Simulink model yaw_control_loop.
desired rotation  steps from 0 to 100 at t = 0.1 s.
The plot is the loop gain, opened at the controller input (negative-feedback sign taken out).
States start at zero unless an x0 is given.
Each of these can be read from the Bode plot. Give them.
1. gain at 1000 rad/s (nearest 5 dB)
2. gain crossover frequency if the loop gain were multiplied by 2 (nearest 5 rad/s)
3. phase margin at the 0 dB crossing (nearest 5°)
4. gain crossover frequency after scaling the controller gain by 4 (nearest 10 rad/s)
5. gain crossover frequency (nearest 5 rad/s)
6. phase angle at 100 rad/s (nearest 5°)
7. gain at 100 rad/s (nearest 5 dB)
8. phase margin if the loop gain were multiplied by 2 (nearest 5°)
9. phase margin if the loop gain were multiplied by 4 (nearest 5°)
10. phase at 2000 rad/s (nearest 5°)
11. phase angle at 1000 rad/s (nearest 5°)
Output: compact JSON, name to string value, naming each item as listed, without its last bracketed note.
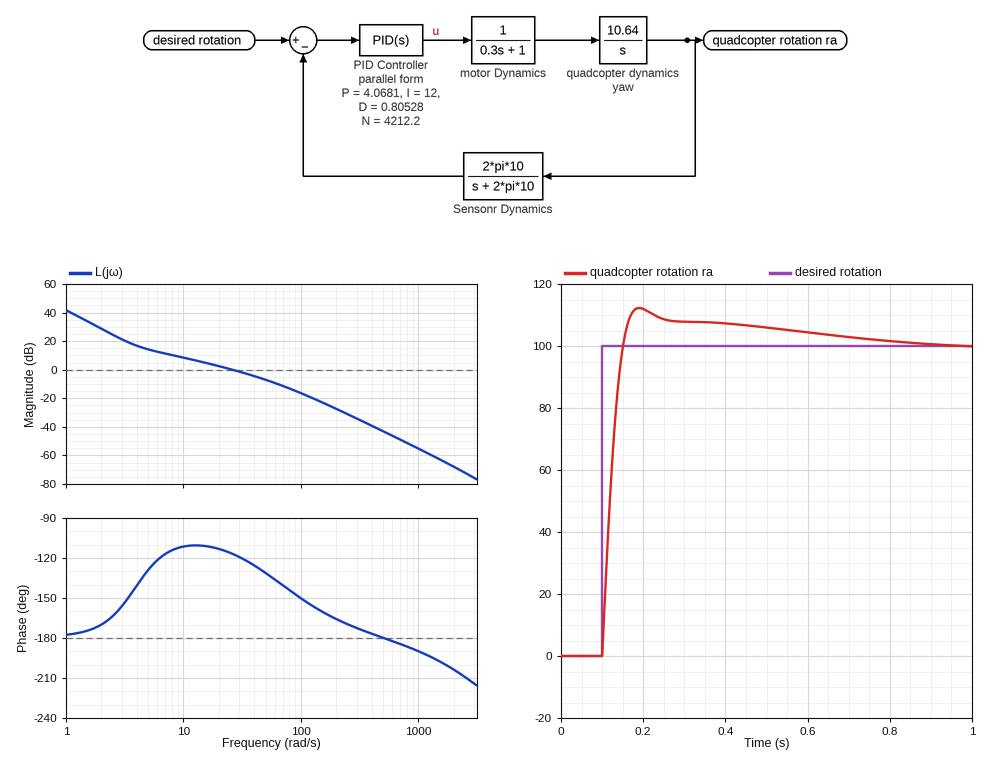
{"gain at 1000 rad/s": "-55 dB", "gain crossover frequency if the loop gain were multiplied by 2": "45 rad/s", "phase margin at the 0 dB crossing": "65°", "gain crossover frequency after scaling the controller gain by 4": "70 rad/s", "gain crossover frequency": "25 rad/s", "phase angle at 100 rad/s": "-150°", "gain at 100 rad/s": "-15 dB", "phase margin if the loop gain were multiplied by 2": "50°", "phase margin if the loop gain were multiplied by 4": "40°", "phase at 2000 rad/s": "-205°", "phase angle at 1000 rad/s": "-190°"}
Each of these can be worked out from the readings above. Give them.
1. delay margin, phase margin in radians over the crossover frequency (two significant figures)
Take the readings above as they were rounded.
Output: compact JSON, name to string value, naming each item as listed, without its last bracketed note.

{"delay margin, phase margin in radians over the crossover frequency": "0.045 s"}
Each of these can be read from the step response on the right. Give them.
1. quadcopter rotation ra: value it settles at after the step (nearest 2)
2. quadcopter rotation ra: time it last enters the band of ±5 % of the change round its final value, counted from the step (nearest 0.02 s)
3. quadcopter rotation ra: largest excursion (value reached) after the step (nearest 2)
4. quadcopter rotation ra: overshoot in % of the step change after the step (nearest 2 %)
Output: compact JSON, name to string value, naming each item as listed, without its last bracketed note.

{"quadcopter rotation ra: value it settles at after the step": "100", "quadcopter rotation ra: time it last enters the band of ±5 % of the change round its final value, counted from the step": "0.46 s", "quadcopter rotation ra: largest excursion (value reached) after the step": "112", "quadcopter rotation ra: overshoot in % of the step change after the step": "12 %"}
